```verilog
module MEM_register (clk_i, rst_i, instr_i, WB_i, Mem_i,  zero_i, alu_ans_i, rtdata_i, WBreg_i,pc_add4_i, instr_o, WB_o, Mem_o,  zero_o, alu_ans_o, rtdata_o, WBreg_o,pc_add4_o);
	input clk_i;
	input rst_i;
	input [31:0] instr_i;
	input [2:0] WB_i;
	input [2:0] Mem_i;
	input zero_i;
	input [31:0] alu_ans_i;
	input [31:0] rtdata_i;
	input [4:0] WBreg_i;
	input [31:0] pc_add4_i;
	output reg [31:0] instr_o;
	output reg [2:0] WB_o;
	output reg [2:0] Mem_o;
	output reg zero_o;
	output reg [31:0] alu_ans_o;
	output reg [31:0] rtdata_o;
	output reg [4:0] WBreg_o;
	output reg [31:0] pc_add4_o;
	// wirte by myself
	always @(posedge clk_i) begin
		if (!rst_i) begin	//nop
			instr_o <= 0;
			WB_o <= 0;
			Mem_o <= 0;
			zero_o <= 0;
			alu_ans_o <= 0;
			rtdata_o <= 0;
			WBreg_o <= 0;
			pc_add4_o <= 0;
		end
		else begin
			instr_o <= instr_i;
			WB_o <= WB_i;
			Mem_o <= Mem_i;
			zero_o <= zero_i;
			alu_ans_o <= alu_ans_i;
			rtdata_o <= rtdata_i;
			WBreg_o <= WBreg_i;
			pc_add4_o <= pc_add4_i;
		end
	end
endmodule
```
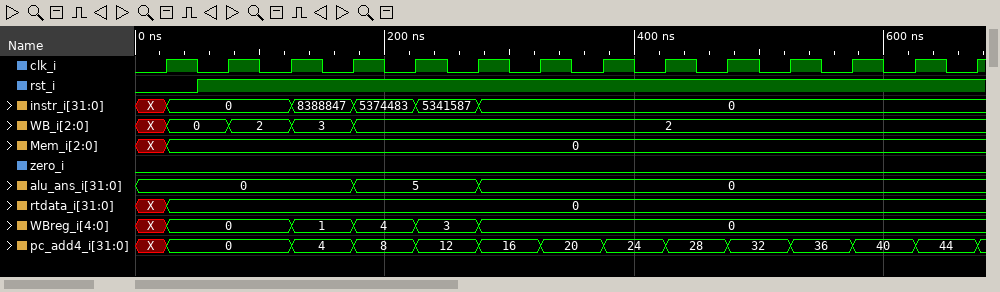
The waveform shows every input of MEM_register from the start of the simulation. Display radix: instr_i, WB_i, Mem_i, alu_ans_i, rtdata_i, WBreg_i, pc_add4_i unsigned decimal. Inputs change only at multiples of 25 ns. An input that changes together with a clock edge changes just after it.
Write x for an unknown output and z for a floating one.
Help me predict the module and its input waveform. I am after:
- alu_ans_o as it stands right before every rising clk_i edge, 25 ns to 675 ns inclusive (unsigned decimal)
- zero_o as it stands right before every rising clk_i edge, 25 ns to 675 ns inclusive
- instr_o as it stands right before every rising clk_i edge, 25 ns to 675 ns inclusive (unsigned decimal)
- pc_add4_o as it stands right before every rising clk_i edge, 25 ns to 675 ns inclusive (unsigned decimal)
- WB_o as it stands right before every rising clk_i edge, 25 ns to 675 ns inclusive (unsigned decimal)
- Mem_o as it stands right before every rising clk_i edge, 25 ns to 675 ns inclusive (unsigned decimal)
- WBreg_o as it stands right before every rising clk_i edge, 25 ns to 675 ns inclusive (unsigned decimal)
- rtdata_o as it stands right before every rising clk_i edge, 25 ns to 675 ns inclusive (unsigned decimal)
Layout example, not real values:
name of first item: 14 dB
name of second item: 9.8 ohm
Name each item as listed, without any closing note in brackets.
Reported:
alu_ans_o as it stands right before every rising clk_i edge, 25 ns to 675 ns inclusive: x, 0, 0, 0, 0, 5, 5, 0, 0, 0, 0, 0, 0, 0
zero_o as it stands right before every rising clk_i edge, 25 ns to 675 ns inclusive: x 0 0 0 0 0 0 0 0 0 0 0 0 0
instr_o as it stands right before every rising clk_i edge, 25 ns to 675 ns inclusive: x, 0, 0, 0, 8388847, 5374483, 5341587, 0, 0, 0, 0, 0, 0, 0
pc_add4_o as it stands right before every rising clk_i edge, 25 ns to 675 ns inclusive: x, 0, 0, 0, 4, 8, 12, 16, 20, 24, 28, 32, 36, 40
WB_o as it stands right before every rising clk_i edge, 25 ns to 675 ns inclusive: x, 0, 0, 2, 3, 2, 2, 2, 2, 2, 2, 2, 2, 2
Mem_o as it stands right before every rising clk_i edge, 25 ns to 675 ns inclusive: x, 0, 0, 0, 0, 0, 0, 0, 0, 0, 0, 0, 0, 0
WBreg_o as it stands right before every rising clk_i edge, 25 ns to 675 ns inclusive: x, 0, 0, 0, 1, 4, 3, 0, 0, 0, 0, 0, 0, 0
rtdata_o as it stands right before every rising clk_i edge, 25 ns to 675 ns inclusive: x, 0, 0, 0, 0, 0, 0, 0, 0, 0, 0, 0, 0, 0
